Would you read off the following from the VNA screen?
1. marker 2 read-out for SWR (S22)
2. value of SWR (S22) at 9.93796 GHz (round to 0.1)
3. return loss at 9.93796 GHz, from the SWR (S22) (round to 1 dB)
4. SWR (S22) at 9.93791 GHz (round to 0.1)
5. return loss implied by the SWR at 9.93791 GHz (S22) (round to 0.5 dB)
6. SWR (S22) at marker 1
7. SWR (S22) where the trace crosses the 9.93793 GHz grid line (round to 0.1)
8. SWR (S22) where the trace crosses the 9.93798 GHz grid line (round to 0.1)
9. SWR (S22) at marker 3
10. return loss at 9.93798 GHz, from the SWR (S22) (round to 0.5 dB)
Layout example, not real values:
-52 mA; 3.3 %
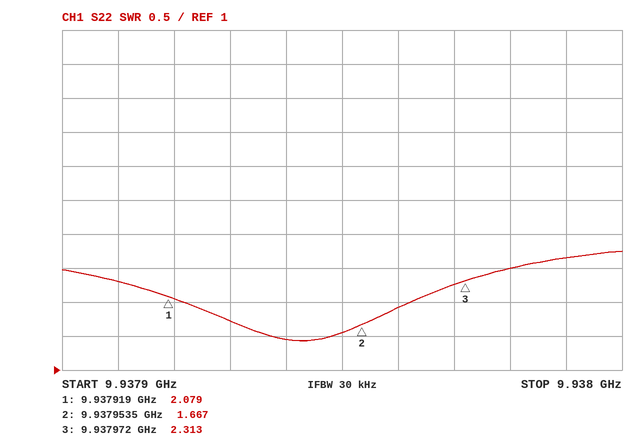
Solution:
1.667; 1.9; 10 dB; 2.3; 8.0 dB; 2.079; 1.7; 2.5; 2.313; 7.5 dB
